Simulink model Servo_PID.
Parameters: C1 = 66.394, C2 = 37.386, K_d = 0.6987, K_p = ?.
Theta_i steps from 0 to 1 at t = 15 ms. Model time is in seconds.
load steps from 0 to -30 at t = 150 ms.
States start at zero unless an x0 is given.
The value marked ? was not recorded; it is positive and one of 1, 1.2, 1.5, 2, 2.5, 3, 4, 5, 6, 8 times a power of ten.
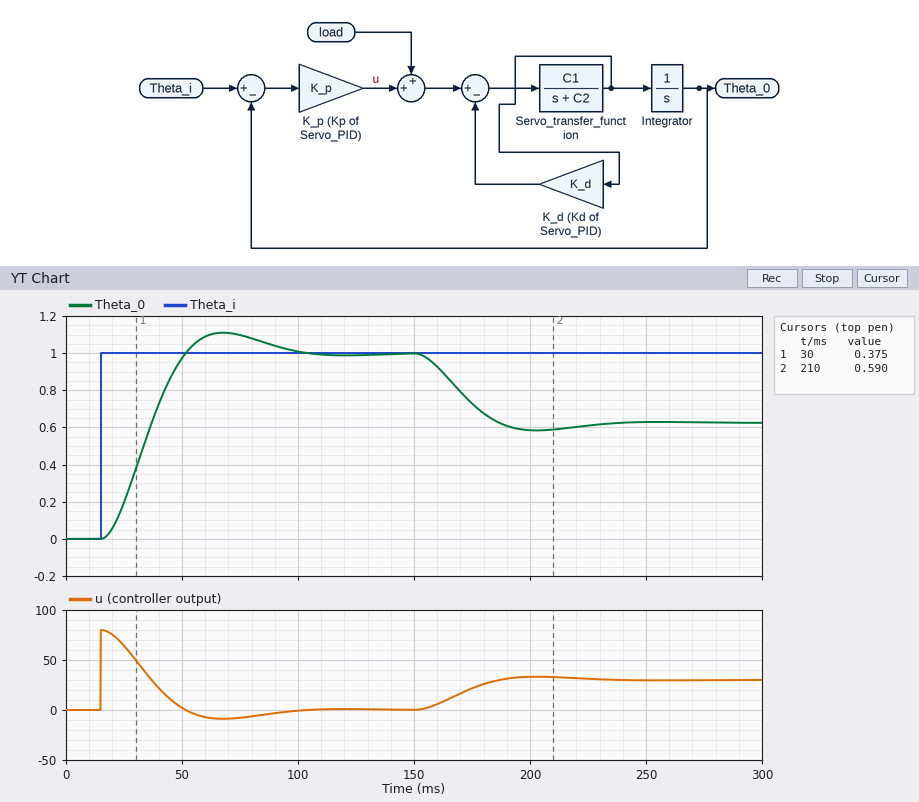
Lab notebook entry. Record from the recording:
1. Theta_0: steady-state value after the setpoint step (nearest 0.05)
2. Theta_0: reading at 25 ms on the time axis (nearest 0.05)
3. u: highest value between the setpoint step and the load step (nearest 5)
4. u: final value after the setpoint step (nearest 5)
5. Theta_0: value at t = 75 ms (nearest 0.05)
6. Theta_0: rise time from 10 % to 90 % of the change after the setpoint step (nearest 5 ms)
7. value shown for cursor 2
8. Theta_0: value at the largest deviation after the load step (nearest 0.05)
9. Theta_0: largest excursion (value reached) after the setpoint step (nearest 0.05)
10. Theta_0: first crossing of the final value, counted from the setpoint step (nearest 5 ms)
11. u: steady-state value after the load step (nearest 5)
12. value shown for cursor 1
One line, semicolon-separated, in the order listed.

1.00; 0.20; 80; 0; 1.10; 25 ms; 0.590; 0.60; 1.10; 35 ms; 30; 0.375
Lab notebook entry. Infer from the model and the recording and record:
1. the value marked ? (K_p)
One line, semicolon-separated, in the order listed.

80
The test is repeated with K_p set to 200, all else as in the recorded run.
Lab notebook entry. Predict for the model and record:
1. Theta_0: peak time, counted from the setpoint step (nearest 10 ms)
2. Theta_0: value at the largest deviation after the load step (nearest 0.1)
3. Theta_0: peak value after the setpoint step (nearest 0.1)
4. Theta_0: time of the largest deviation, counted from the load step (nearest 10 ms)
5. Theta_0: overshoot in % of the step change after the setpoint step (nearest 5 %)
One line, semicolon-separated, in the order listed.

30 ms; 0.8; 1.3; 30 ms; 30 %
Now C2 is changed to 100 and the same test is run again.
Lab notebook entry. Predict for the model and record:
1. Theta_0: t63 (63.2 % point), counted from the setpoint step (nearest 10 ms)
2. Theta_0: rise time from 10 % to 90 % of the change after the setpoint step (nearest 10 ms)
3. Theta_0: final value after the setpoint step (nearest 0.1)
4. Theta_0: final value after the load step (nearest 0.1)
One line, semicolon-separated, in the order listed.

30 ms; 50 ms; 1.0; 0.6
